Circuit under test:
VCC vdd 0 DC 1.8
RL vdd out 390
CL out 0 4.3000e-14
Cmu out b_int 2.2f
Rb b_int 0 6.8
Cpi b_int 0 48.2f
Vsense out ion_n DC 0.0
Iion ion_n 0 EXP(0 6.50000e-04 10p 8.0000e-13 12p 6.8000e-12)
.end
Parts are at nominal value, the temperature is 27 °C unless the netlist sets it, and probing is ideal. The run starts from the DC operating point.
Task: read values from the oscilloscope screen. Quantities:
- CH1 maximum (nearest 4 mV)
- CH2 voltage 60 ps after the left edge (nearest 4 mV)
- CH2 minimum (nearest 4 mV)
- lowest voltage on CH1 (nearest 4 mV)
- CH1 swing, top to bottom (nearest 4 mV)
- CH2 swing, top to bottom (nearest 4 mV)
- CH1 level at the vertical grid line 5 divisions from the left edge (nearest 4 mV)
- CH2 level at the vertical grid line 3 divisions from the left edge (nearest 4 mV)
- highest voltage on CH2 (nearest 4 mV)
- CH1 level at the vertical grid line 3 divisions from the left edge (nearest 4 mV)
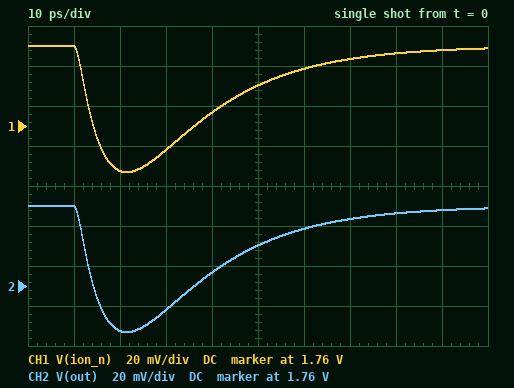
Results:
1.800 V
1.788 V
1.736 V
1.736 V
64 mV
64 mV
1.780 V
1.748 V
1.800 V
1.748 V
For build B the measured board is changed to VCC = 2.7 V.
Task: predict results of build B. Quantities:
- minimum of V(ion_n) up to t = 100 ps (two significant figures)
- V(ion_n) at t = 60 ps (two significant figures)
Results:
2.6 V
2.7 V
